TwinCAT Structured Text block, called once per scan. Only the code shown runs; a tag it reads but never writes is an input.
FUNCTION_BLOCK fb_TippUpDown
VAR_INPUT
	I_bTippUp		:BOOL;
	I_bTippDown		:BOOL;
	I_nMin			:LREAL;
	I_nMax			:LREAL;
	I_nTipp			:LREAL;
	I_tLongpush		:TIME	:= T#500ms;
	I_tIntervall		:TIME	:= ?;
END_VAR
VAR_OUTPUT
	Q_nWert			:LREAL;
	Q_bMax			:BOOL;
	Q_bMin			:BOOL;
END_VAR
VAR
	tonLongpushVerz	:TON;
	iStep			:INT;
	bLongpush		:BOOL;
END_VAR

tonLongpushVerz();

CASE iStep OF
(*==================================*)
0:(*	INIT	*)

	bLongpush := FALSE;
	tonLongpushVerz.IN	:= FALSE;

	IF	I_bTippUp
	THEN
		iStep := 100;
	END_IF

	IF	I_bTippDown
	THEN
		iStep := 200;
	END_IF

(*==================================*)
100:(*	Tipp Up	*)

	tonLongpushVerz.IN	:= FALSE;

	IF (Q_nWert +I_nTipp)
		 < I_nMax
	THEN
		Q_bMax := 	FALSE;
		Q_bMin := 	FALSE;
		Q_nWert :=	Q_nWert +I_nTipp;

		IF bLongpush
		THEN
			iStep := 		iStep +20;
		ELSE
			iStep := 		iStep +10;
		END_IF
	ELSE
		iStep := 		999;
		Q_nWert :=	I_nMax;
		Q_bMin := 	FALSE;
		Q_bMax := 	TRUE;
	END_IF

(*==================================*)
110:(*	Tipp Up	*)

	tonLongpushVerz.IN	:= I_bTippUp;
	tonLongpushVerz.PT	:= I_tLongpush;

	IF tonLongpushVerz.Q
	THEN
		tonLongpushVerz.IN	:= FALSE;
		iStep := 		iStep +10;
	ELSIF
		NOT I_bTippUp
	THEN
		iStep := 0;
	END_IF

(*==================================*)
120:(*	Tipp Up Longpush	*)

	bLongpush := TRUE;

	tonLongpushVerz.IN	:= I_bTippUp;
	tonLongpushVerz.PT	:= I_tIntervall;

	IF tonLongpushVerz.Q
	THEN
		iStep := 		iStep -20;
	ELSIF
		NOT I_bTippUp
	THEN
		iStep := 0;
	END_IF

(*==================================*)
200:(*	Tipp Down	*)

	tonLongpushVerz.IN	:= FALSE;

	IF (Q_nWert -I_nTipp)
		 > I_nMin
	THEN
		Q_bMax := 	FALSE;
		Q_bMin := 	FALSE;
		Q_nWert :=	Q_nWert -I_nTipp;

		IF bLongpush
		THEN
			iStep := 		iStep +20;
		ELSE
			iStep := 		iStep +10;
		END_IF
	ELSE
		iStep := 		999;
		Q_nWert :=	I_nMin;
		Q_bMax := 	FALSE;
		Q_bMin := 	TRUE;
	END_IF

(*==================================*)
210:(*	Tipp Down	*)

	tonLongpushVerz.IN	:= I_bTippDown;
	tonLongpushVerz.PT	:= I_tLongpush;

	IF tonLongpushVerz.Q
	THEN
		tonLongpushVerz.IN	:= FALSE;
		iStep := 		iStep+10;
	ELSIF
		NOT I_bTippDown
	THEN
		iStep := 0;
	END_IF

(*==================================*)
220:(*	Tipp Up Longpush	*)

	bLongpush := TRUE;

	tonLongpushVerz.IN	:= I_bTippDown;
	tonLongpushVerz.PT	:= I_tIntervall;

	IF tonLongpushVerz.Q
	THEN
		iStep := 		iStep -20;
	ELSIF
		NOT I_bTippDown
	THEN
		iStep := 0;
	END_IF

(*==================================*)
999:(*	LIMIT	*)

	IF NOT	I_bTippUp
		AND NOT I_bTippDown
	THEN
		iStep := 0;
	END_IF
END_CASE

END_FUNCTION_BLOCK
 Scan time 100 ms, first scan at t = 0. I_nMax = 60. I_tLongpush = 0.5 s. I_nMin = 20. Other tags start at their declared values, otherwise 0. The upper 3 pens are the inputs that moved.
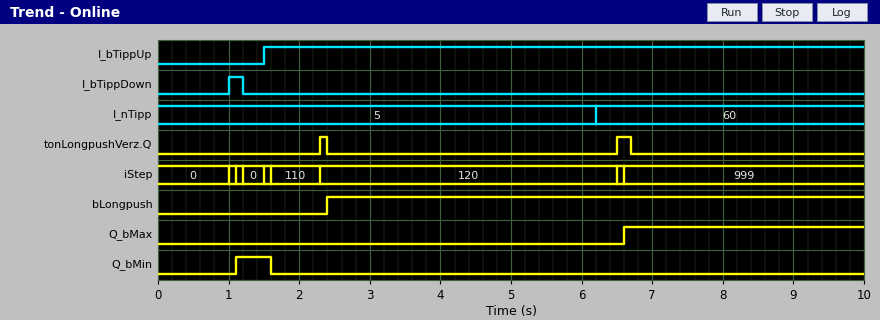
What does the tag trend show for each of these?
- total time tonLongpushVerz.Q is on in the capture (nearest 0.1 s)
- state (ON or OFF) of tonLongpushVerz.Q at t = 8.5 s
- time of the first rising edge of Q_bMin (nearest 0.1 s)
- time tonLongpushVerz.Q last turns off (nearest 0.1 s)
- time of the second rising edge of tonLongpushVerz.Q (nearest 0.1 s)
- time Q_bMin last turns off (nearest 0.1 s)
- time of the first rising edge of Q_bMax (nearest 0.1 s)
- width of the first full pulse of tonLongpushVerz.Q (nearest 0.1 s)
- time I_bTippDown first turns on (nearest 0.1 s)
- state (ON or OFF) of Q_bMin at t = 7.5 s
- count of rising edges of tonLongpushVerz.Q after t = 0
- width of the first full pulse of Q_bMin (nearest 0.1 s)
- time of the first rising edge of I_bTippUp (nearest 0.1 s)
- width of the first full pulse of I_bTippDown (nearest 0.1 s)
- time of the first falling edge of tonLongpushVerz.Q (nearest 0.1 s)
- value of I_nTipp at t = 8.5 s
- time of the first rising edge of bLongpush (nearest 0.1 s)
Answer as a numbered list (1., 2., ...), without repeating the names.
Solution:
1. 0.3 s
2. OFF
3. 1.1 s
4. 6.7 s
5. 6.5 s
6. 1.6 s
7. 6.6 s
8. 0.1 s
9. 1.0 s
10. OFF
11. 2
12. 0.5 s
13. 1.5 s
14. 0.2 s
15. 2.4 s
16. 60
17. 2.4 s
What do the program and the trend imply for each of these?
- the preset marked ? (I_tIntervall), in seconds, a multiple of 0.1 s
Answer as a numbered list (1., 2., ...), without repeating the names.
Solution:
1. 4.0 s
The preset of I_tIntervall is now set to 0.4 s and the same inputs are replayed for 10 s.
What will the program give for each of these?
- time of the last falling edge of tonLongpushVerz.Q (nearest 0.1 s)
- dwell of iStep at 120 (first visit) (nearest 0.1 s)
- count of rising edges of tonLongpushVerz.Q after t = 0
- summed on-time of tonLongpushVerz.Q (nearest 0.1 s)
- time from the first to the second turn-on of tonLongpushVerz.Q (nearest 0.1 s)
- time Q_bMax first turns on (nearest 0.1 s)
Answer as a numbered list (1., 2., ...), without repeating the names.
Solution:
1. 6.6 s
2. 0.6 s
3. 7
4. 1.3 s
5. 0.6 s
6. 6.5 s
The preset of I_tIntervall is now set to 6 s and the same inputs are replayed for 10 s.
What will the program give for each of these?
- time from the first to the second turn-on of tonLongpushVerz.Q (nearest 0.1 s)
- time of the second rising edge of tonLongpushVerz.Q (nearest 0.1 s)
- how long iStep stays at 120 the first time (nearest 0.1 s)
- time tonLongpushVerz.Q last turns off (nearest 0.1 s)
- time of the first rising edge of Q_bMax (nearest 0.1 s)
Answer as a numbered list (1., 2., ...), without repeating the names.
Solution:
1. 6.2 s
2. 8.5 s
3. 6.2 s
4. 8.7 s
5. 8.6 s
